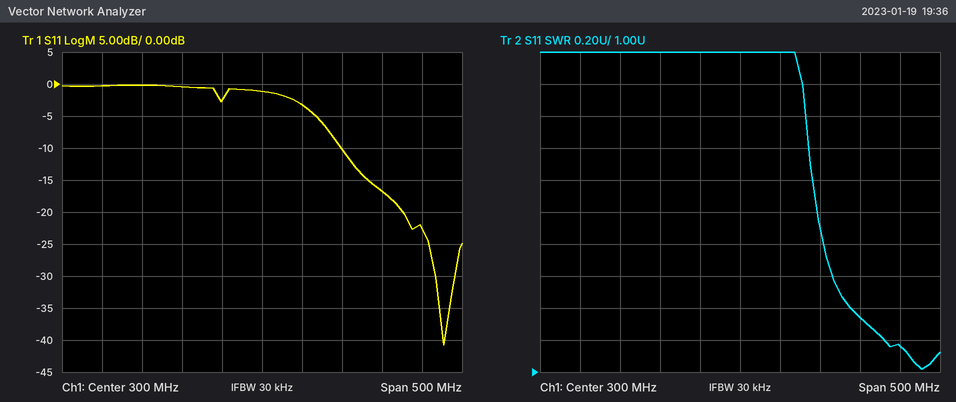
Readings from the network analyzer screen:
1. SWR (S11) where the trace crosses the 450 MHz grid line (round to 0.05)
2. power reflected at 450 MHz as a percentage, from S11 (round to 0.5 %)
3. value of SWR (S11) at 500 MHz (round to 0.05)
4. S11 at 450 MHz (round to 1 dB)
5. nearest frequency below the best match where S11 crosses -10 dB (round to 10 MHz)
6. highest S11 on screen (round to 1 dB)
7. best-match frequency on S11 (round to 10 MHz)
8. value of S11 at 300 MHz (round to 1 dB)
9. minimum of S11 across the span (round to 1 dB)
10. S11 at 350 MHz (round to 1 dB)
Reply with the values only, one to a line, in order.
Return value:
1.35
2.0 %
1.15
-17 dB
400 MHz
0 dB
530 MHz
-1 dB
-41 dB
-3 dB
